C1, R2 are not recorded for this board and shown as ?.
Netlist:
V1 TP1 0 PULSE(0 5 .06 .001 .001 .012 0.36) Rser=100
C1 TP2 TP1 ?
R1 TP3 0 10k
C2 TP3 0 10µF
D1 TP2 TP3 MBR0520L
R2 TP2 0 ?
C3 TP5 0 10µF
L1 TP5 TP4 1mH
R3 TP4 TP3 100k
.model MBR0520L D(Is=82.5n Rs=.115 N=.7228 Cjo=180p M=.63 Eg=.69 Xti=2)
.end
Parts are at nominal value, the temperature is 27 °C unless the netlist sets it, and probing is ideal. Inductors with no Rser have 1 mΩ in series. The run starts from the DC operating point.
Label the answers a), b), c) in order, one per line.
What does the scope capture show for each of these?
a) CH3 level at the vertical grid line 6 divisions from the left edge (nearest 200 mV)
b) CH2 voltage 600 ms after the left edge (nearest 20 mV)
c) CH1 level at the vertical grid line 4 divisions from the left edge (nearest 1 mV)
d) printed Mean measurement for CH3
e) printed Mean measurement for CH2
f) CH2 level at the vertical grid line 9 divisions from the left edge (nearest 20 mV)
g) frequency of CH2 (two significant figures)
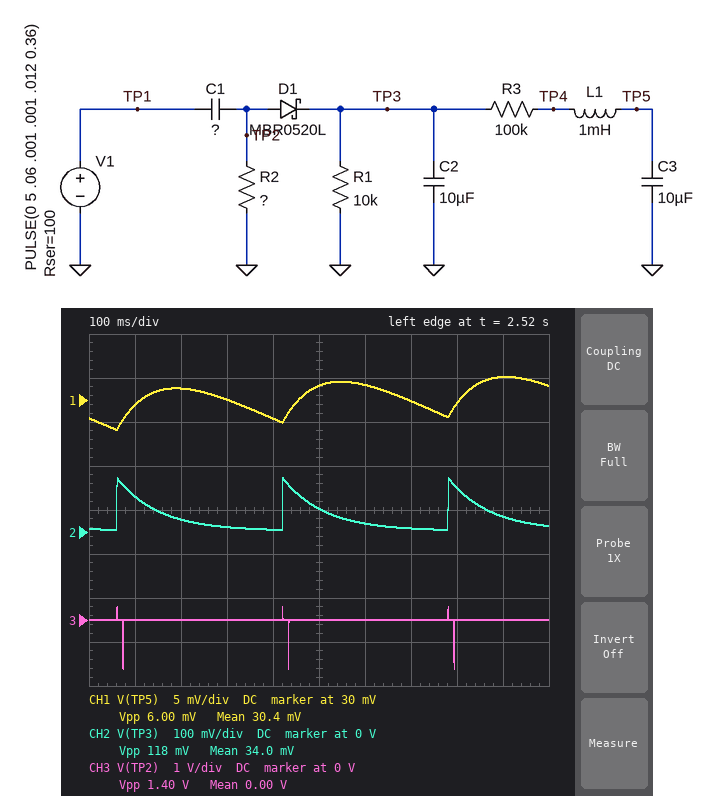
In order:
a) 0 V
b) 20 mV
c) 28 mV
d) 0.00 V
e) 34.0 mV
f) 40 mV
g) 2.8 Hz
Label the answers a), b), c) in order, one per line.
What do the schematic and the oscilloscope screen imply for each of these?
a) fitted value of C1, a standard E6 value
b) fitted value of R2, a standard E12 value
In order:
a) 330 nF
b) 680 Ω
